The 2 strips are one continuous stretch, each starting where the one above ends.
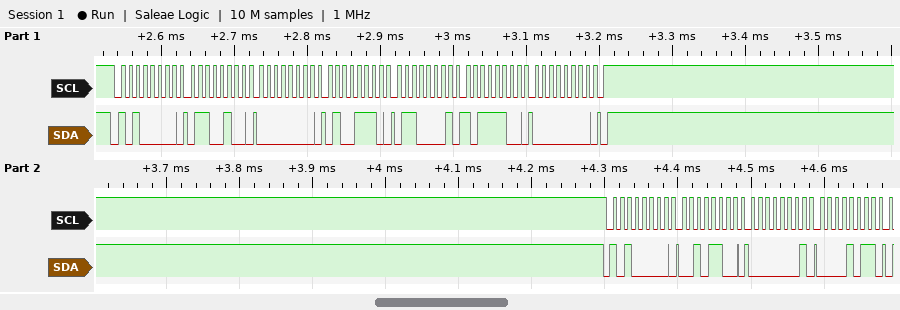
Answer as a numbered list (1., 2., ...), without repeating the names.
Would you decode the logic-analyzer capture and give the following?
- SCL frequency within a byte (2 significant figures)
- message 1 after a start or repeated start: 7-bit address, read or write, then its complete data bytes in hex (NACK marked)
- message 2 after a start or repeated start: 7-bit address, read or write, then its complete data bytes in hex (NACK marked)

1. 100 kHz
2. 0x50 write: 64 00 4E 61 BC 00
3. 0x50 write: 2C 01 0B
